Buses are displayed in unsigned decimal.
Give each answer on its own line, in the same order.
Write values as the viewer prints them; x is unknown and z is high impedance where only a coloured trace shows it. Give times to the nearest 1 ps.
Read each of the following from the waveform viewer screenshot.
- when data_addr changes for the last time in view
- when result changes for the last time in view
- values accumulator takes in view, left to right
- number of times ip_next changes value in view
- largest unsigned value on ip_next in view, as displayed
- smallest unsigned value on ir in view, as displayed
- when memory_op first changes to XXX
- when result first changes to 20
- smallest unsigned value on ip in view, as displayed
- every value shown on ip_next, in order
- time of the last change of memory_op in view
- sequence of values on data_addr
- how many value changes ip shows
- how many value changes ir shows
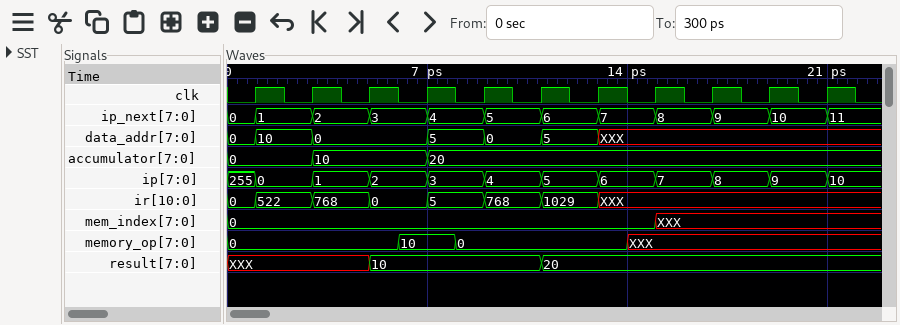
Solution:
13 ps
11 ps
0, 10, 20
11
11
0
14 ps
11 ps
0
0, 1, 2, 3, 4, 5, 6, 7, 8, 9, 10, 11
14 ps
0, 10, 0, 5, 0, 5, XXX
11
7
